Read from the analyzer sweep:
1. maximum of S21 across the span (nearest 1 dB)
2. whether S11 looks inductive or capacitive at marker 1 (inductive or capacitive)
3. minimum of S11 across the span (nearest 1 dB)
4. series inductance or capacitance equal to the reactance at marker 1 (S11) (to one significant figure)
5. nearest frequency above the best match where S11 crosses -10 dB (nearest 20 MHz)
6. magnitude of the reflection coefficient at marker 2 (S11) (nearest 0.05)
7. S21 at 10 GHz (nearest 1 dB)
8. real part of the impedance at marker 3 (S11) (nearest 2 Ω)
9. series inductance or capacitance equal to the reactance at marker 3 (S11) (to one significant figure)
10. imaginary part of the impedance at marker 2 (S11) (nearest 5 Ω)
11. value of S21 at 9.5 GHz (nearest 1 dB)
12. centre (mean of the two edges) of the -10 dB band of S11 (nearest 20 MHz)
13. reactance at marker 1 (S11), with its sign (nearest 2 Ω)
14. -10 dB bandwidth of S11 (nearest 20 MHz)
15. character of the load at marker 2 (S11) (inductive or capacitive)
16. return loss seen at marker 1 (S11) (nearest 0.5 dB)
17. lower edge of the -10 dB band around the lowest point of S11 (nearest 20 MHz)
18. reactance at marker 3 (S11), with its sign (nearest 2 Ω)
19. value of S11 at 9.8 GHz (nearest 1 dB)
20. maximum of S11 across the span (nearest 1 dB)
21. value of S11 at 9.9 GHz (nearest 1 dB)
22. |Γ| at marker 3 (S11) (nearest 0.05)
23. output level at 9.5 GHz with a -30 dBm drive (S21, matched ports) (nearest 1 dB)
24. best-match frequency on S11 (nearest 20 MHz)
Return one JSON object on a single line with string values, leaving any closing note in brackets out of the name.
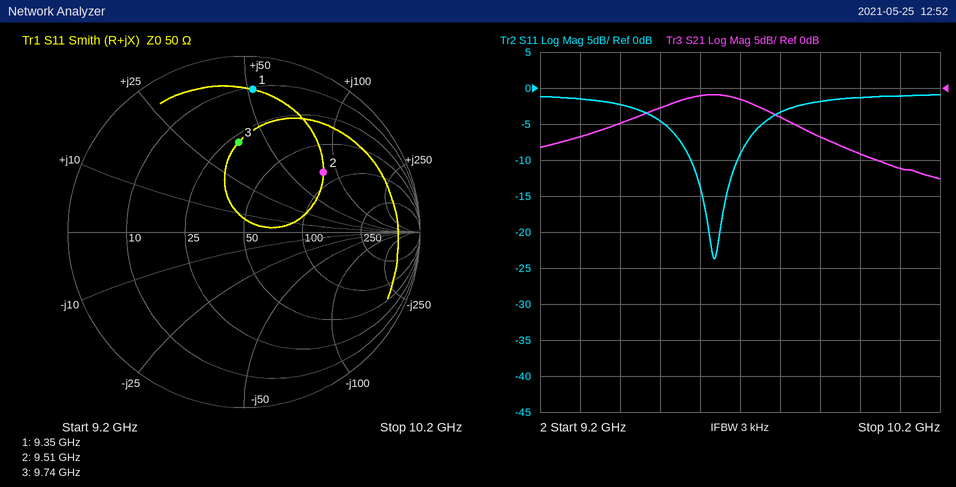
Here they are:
{"maximum of S21 across the span": "-1 dB", "whether S11 looks inductive or capacitive at marker 1": "inductive", "minimum of S11 across the span": "-24 dB", "series inductance or capacitance equal to the reactance at marker 1 (S11)": "900 pH", "nearest frequency above the best match where S11 crosses -10 dB": "9.70 GHz", "magnitude of the reflection coefficient at marker 2 (S11)": "0.55", "S21 at 10 GHz": "-9 dB", "real part of the impedance at marker 3 (S11)": "28 Ω", "series inductance or capacitance equal to the reactance at marker 3 (S11)": "600 pH", "imaginary part of the impedance at marker 2 (S11)": "+80 Ω", "value of S21 at 9.5 GHz": "-3 dB", "centre (mean of the two edges) of the -10 dB band of S11": "9.64 GHz", "reactance at marker 1 (S11), with its sign": "+52 Ω", "-10 dB bandwidth of S11": "120 MHz", "character of the load at marker 2 (S11)": "inductive", "return loss seen at marker 1 (S11)": "2.0 dB", "lower edge of the -10 dB band around the lowest point of S11": "9.58 GHz", "reactance at marker 3 (S11), with its sign": "+38 Ω", "value of S11 at 9.8 GHz": "-3 dB", "maximum of S11 across the span": "-1 dB", "value of S11 at 9.9 GHz": "-2 dB", "|Γ| at marker 3 (S11)": "0.50", "output level at 9.5 GHz with a -30 dBm drive (S21, matched ports)": "-33 dBm", "best-match frequency on S11": "9.64 GHz"}
